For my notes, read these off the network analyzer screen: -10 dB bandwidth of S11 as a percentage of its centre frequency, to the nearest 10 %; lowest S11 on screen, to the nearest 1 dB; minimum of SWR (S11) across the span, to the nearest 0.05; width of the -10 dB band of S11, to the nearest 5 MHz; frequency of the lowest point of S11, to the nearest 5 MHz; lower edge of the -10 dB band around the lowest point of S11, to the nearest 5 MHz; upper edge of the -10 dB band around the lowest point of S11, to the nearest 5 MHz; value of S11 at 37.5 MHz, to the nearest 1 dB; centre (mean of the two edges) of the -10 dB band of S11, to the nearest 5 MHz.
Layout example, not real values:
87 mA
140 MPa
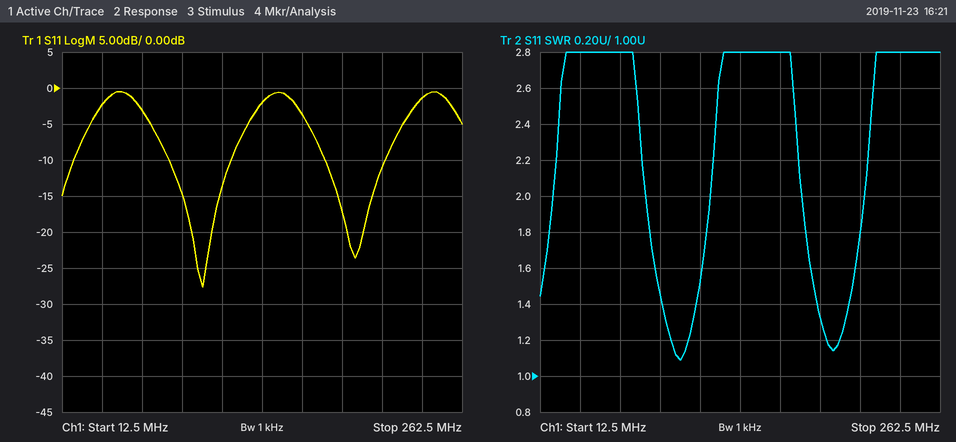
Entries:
40 %
-28 dB
1.10
40 MHz
100 MHz
80 MHz
120 MHz
-2 dB
100 MHz
